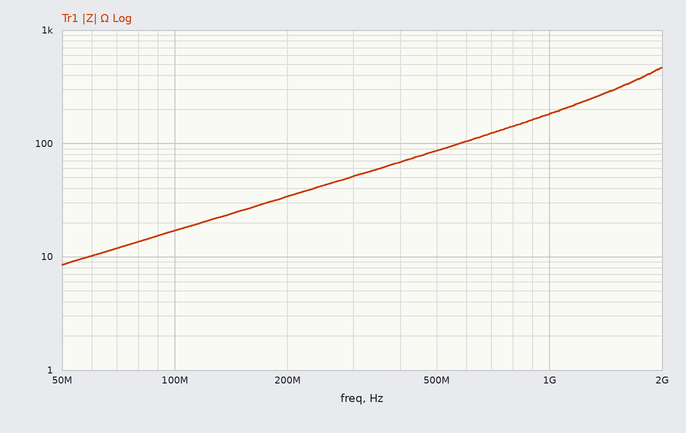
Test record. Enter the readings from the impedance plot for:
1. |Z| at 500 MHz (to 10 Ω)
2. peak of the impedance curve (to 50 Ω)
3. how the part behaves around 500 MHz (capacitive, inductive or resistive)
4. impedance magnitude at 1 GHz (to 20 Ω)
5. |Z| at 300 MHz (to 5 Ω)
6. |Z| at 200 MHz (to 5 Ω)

90 Ω
450 Ω
inductive
180 Ω
50 Ω
35 Ω
